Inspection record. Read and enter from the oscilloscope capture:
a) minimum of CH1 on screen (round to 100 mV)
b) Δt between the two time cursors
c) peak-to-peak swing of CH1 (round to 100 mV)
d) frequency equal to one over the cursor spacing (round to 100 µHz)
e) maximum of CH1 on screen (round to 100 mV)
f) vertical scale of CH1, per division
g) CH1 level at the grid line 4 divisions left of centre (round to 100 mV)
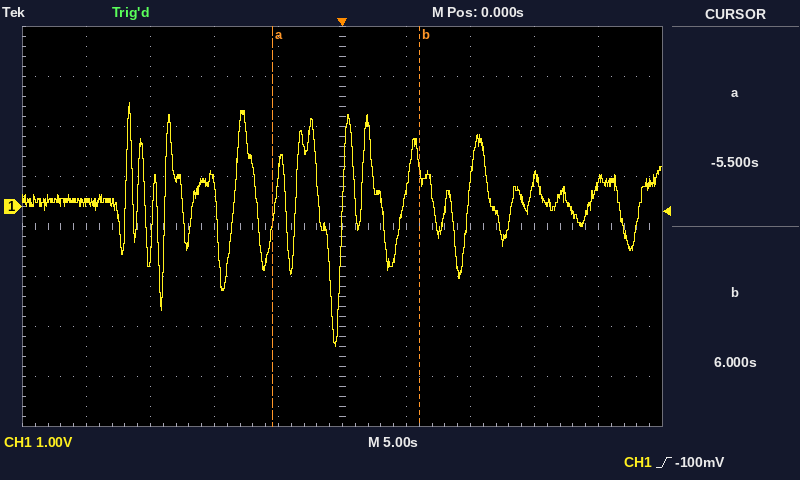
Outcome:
-2.8 V
11.5 s
4.9 V
87.0 mHz
2.1 V
1 V
100 mV
